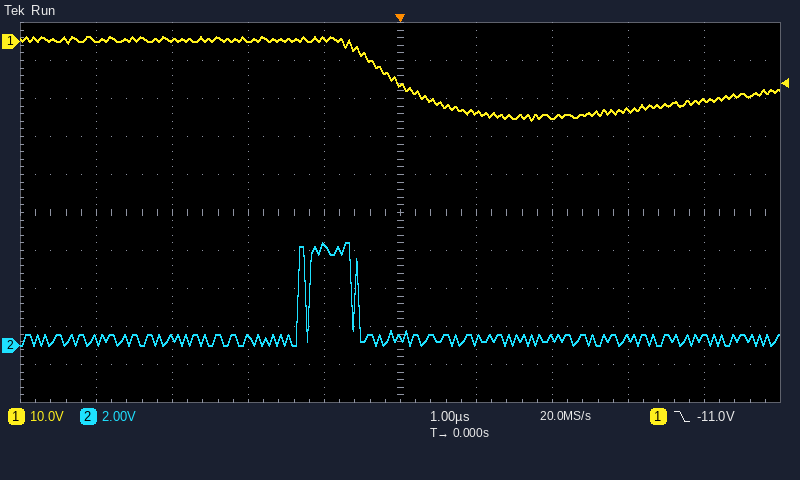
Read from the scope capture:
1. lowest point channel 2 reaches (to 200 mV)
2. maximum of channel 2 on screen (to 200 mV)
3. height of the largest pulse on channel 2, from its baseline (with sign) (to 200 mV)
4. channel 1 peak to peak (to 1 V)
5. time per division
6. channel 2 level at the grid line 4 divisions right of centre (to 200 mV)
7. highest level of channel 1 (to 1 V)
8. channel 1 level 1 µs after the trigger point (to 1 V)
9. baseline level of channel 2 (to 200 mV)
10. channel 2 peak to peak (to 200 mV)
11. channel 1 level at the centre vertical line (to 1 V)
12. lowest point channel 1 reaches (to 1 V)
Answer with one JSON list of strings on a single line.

["0.0 V", "5.4 V", "+5.0 V", "22 V", "1 µs", "400 mV", "1 V", "-19 V", "400 mV", "5.4 V", "-11 V", "-21 V"]
